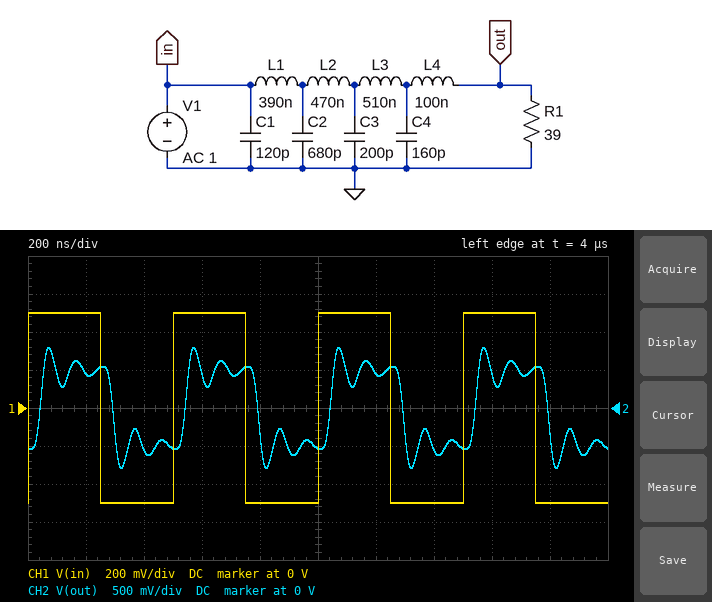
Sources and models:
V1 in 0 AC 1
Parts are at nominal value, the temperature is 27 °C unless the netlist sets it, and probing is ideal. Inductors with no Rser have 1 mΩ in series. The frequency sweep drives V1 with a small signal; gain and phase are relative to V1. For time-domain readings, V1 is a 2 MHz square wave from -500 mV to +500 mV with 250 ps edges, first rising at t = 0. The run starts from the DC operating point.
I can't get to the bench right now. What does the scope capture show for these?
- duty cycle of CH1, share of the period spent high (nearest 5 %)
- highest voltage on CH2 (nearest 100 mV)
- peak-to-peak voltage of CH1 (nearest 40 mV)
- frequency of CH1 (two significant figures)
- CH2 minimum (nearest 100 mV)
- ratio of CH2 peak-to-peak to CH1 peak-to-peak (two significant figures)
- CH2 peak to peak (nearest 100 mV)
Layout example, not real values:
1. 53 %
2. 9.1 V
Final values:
1. 50 %
2. 800 mV
3. 1.00 V
4. 2.0 MHz
5. -800 mV
6. 1.6
7. 1.6 V
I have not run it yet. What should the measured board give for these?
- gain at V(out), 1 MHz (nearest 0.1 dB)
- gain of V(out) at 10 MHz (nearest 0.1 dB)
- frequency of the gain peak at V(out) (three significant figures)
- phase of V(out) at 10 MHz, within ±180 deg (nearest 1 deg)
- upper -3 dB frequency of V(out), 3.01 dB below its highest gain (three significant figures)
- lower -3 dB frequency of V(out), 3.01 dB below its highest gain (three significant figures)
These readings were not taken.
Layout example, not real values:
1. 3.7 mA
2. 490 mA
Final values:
1. 0 dB
2. 5.7 dB
3. 10.5 MHz
4. -152 deg
5. 12.1 MHz
6. 8.19 MHz
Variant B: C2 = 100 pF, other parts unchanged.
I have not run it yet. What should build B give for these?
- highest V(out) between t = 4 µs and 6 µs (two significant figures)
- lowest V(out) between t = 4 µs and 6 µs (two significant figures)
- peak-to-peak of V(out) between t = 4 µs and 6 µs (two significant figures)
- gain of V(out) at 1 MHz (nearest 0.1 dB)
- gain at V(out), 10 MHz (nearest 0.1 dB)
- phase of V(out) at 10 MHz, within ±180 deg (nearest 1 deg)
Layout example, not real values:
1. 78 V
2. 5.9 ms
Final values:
1. 520 mV
2. -520 mV
3. 1.0 V
4. -0.1 dB
5. -3.2 dB
6. -104 deg
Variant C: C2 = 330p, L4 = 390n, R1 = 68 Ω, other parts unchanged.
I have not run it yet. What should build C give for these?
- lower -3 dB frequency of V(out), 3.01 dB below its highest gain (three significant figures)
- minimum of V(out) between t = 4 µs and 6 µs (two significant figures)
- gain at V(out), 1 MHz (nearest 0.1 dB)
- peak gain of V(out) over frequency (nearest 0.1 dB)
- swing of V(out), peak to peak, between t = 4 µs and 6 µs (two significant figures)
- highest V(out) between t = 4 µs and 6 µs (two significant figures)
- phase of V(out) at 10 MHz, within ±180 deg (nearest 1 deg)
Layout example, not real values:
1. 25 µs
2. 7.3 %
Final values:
1. 5.03 MHz
2. -1.0 V
3. 0.1 dB
4. 4.7 dB
5. 2.0 V
6. 1.0 V
7. -132 deg
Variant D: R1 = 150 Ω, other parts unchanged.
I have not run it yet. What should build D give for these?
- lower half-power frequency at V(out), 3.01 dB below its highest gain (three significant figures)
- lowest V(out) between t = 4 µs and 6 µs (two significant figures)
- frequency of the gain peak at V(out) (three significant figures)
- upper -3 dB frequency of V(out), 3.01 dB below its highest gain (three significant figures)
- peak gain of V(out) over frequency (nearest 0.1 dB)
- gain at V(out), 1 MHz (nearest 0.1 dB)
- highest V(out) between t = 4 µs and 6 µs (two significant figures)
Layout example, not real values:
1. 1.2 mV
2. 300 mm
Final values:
1. 6.13 MHz
2. -1.6 V
3. 7.23 MHz
4. 8.45 MHz
5. 13.3 dB
6. 0.2 dB
7. 1.6 V
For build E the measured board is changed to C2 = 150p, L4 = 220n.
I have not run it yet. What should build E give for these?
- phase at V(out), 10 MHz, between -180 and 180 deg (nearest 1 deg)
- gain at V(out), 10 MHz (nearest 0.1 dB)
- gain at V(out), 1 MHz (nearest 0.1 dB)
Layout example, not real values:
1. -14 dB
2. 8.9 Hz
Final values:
1. -106 deg
2. -2.1 dB
3. -0.1 dB
